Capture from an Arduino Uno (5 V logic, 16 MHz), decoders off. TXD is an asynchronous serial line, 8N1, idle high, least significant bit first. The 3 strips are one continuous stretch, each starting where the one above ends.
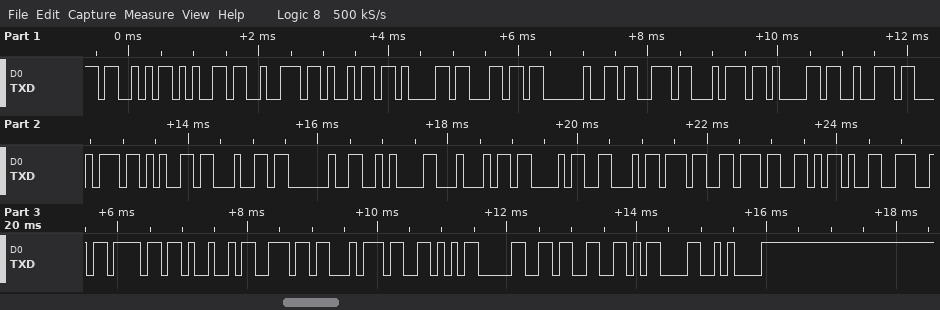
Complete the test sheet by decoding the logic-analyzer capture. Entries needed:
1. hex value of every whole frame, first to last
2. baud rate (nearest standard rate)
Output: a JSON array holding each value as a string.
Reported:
["53 65 72 69 61 6C 20 73 74 61 72 74 65 64 20 0A 44 43 46 37 37 2D 4E 6F 49 6E 74 56 30 33 0D 0A", "9600 baud"]
